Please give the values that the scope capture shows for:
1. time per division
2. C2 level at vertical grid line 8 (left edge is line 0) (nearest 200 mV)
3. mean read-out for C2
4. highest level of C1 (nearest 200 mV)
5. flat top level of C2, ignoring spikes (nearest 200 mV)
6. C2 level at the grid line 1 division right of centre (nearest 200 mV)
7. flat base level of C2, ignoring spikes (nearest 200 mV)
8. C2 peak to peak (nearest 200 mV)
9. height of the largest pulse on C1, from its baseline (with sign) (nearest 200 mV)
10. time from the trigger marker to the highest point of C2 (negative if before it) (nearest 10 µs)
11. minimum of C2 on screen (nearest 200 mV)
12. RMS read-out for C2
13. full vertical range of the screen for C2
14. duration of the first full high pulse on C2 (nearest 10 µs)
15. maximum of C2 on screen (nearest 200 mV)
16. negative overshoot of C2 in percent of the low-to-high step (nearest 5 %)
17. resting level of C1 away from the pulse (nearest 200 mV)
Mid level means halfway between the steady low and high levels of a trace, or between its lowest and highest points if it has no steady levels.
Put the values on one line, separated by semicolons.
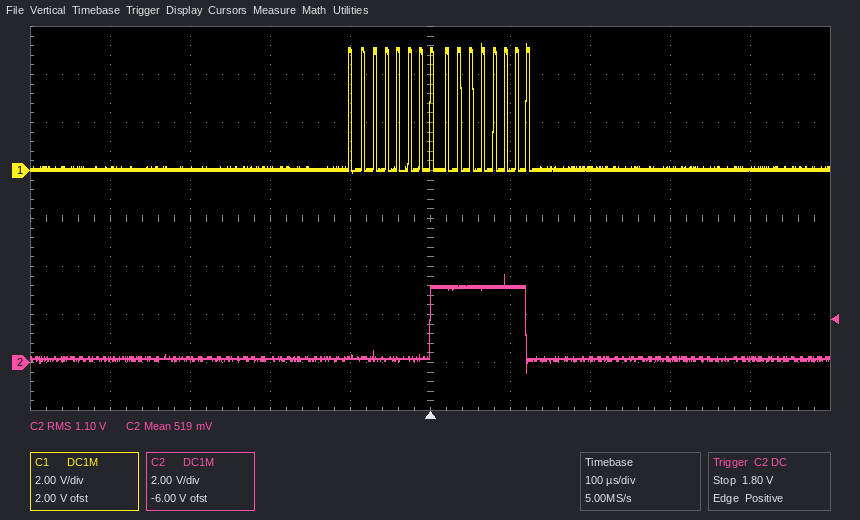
100 µs; 200 mV; 519 mV; 5.2 V; 3.2 V; 3.2 V; 200 mV; 4.0 V; +5.2 V; +90 µs; -400 mV; 1.10 V; 16 V; 120 µs; 3.6 V; 20 %; 0.0 V
